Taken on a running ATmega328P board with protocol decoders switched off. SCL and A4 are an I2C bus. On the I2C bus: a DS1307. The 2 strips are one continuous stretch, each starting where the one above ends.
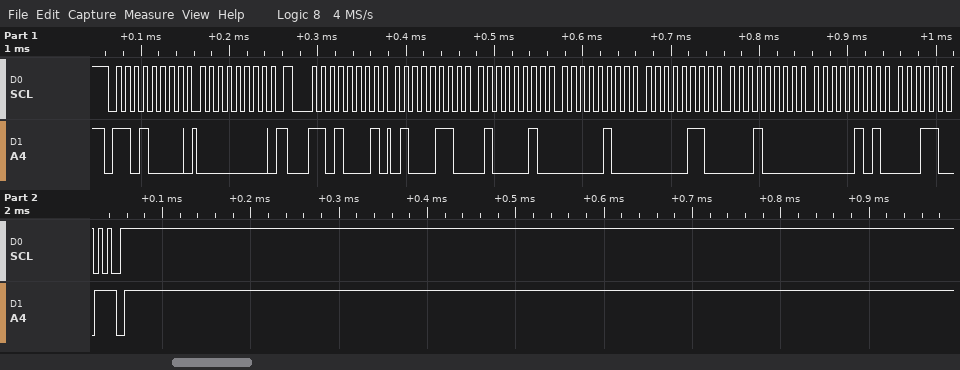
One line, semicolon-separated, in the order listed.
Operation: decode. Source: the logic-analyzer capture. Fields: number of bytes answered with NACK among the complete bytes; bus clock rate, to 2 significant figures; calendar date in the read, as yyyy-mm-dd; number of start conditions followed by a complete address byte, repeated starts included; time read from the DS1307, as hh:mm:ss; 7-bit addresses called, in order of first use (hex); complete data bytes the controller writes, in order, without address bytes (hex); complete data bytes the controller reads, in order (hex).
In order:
1; 100 kHz; 2019-05-10; 2; 04:42:46; 0x68; 00; 46 42 04 06 10 05 19
